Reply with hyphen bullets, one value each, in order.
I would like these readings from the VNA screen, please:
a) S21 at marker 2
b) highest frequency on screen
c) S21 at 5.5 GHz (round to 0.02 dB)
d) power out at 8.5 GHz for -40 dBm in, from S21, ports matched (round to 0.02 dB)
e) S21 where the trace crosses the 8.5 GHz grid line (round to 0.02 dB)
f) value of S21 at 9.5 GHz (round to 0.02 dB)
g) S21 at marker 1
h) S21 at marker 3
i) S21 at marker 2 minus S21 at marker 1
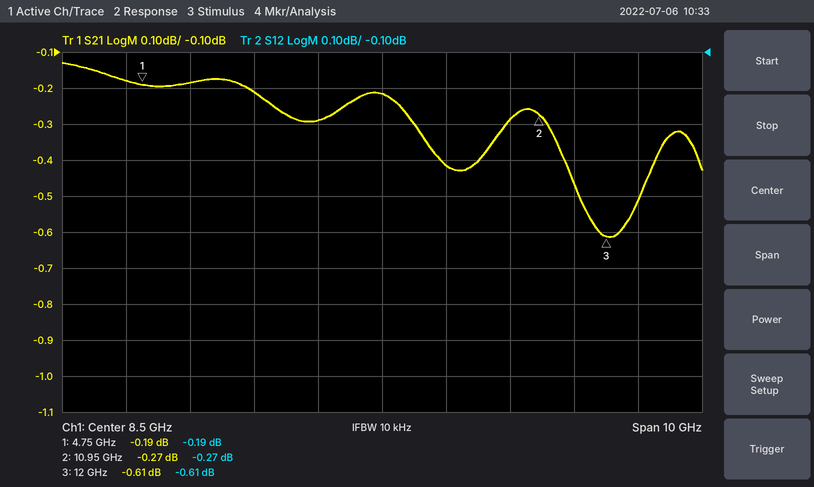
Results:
- -0.27 dB
- 13.5 GHz
- -0.18 dB
- -40.22 dBm
- -0.22 dB
- -0.42 dB
- -0.19 dB
- -0.61 dB
- -0.08 dB
